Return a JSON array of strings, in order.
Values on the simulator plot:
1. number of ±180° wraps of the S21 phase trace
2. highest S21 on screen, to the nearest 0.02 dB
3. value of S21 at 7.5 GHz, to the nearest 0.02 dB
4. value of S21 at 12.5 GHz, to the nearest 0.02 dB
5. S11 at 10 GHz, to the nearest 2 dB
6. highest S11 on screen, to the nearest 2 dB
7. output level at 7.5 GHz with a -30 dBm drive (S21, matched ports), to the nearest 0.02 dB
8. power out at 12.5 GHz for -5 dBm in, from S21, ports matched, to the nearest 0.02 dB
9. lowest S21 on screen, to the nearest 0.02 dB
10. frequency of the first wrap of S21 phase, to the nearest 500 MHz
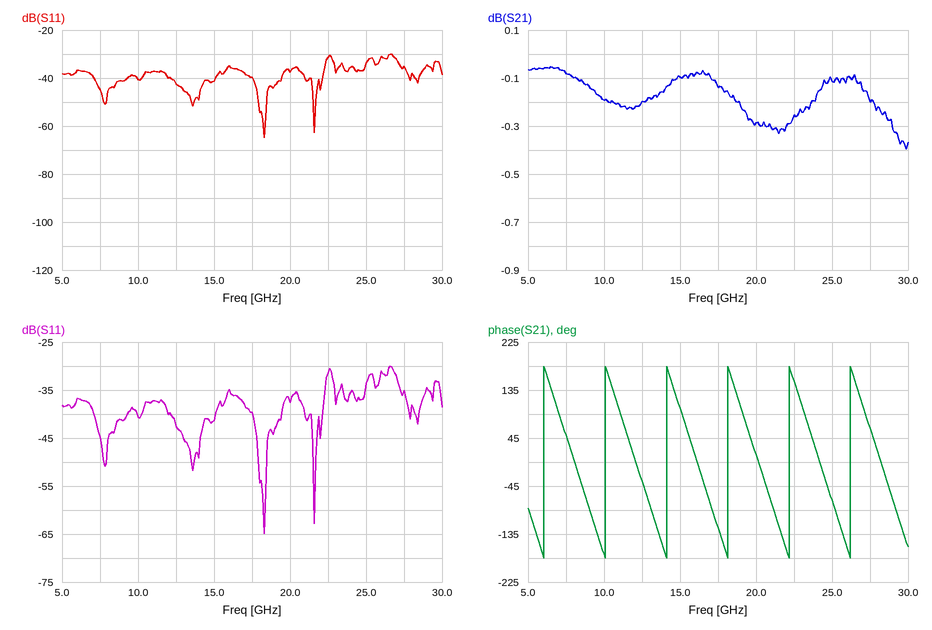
["6", "-0.06 dB", "-0.08 dB", "-0.20 dB", "-40 dB", "-30 dB", "-30.08 dBm", "-5.20 dBm", "-0.40 dB", "6.0 GHz"]
